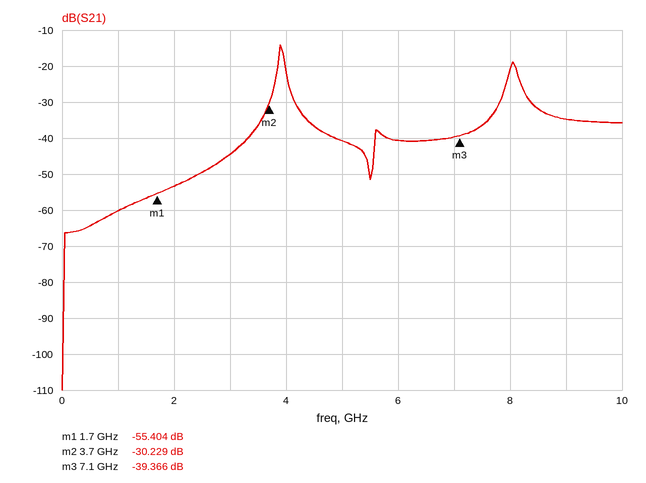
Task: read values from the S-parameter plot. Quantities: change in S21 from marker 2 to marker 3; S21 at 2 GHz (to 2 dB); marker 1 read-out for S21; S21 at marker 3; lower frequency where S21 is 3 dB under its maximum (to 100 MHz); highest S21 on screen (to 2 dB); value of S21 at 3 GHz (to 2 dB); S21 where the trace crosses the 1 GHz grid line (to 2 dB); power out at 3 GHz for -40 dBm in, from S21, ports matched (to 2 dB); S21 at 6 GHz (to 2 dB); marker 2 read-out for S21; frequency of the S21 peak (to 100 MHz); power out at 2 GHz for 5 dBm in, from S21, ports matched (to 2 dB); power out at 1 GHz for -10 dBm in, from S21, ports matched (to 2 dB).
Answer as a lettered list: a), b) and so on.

a) -9.137 dB
b) -54 dB
c) -55.404 dB
d) -39.366 dB
e) 3.9 GHz
f) -14 dB
g) -44 dB
h) -60 dB
i) -84 dBm
j) -40 dB
k) -30.229 dB
l) 3.9 GHz
m) -48 dBm
n) -70 dBm
